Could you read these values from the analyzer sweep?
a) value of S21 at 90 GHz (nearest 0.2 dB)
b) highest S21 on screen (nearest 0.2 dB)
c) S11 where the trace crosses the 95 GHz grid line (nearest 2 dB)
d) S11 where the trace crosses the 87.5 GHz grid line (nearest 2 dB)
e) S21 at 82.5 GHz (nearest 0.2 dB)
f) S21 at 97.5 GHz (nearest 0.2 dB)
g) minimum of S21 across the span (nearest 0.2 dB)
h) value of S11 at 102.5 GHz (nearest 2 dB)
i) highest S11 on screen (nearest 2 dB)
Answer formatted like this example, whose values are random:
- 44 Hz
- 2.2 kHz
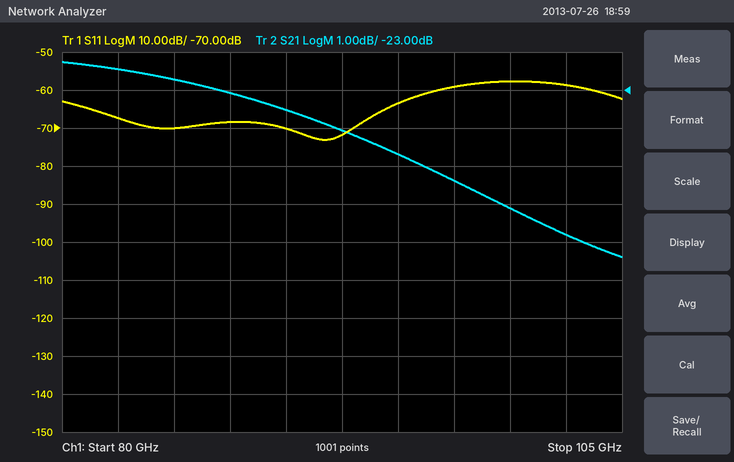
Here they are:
- -23.6 dB
- -22.2 dB
- -64 dB
- -68 dB
- -22.4 dB
- -25.4 dB
- -27.4 dB
- -58 dB
- -58 dB
